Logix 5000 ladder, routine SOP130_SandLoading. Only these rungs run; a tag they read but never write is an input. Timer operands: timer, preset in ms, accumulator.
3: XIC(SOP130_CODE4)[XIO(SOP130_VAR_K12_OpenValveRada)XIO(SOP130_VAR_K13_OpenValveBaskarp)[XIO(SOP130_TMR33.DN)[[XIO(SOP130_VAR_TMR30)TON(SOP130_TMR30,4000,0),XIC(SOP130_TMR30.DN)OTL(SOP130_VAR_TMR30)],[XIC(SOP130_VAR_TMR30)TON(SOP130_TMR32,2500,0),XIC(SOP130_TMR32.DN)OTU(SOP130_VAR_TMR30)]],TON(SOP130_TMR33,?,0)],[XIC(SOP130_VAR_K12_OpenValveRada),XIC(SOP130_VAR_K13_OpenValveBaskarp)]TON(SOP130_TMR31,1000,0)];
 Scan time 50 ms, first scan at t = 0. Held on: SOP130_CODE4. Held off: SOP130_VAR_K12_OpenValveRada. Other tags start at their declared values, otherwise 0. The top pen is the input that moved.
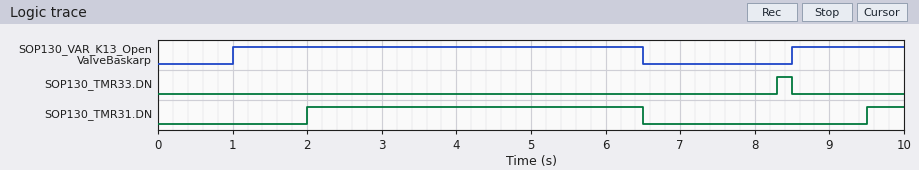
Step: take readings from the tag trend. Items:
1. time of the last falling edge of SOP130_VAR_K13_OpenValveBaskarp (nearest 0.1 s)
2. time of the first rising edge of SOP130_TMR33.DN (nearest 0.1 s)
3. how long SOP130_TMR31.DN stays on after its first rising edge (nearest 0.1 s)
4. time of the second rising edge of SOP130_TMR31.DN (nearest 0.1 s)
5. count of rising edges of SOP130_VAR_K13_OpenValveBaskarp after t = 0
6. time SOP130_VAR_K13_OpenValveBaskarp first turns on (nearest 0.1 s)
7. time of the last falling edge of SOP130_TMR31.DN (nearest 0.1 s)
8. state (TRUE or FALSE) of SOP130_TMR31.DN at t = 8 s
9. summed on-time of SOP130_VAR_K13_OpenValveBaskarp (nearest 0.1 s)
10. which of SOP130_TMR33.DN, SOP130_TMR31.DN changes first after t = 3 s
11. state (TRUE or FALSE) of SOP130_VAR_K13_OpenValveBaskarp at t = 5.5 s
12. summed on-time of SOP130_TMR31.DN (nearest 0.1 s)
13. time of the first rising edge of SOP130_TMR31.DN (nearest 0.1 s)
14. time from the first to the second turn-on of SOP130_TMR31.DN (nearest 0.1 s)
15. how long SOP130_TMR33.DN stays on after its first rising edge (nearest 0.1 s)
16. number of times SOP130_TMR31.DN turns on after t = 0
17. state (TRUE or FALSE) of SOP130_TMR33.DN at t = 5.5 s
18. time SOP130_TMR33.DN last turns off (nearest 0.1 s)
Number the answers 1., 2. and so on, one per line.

1. 6.5 s
2. 8.3 s
3. 4.5 s
4. 9.5 s
5. 2
6. 1.0 s
7. 6.5 s
8. FALSE
9. 7.0 s
10. SOP130_TMR31.DN
11. TRUE
12. 5.0 s
13. 2.0 s
14. 7.5 s
15. 0.2 s
16. 2
17. FALSE
18. 8.5 s
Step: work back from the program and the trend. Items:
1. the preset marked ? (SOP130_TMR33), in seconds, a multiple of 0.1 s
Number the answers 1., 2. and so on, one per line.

1. 1.8 s
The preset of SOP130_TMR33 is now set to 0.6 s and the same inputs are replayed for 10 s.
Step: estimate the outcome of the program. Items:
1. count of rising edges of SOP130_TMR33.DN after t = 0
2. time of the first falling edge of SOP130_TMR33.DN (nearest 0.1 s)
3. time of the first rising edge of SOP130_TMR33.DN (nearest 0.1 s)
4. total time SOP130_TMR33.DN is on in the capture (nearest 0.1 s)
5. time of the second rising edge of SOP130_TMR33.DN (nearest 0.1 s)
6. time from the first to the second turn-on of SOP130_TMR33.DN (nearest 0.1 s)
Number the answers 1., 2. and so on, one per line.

1. 2
2. 1.0 s
3. 0.6 s
4. 1.8 s
5. 7.1 s
6. 6.5 s
